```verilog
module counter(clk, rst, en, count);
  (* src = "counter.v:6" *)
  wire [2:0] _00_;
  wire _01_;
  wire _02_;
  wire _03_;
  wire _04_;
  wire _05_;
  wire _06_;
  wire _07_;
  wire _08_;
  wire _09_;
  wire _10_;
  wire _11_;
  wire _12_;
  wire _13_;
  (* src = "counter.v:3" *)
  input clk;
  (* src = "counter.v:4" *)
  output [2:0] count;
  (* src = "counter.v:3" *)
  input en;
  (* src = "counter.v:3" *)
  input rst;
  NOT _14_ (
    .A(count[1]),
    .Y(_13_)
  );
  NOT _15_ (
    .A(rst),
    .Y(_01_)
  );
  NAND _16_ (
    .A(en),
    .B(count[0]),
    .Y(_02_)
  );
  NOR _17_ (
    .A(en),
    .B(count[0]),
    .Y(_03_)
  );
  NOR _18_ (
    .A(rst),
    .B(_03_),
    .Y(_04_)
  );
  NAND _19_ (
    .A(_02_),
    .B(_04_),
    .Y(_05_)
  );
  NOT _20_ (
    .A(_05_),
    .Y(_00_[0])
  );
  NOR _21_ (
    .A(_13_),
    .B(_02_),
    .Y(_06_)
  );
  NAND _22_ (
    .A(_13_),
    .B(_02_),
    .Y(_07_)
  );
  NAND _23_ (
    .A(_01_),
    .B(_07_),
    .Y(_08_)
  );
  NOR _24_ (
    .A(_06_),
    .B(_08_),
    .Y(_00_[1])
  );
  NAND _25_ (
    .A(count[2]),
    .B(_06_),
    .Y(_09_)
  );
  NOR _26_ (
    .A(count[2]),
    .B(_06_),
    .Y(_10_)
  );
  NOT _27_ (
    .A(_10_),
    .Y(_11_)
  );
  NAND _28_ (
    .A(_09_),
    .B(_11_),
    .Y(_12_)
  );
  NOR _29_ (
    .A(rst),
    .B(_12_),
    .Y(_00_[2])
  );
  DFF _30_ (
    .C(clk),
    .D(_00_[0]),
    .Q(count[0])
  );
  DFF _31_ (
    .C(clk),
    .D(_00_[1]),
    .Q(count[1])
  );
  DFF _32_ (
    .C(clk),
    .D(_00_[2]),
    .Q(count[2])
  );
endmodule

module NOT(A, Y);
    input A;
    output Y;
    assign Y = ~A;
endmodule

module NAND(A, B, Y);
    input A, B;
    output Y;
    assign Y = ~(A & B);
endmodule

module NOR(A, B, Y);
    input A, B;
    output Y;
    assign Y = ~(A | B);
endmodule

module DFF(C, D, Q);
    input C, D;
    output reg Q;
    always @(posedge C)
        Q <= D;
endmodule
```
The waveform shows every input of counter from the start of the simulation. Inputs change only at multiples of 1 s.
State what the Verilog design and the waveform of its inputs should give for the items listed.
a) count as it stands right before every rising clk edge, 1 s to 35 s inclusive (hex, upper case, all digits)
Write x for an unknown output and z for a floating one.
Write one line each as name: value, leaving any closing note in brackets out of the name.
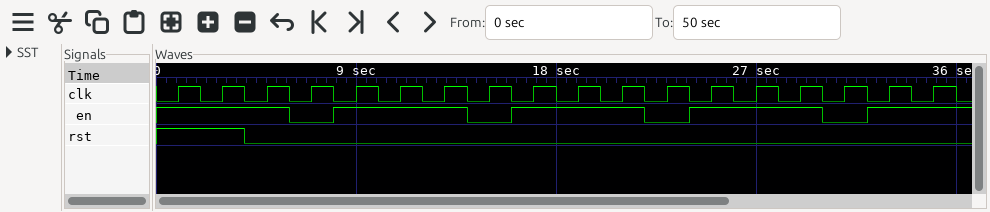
count as it stands right before every rising clk edge, 1 s to 35 s inclusive: x, 0, 0, 1, 1, 2, 3, 4, 4, 5, 6, 7, 7, 0, 1, 2, 2, 3
